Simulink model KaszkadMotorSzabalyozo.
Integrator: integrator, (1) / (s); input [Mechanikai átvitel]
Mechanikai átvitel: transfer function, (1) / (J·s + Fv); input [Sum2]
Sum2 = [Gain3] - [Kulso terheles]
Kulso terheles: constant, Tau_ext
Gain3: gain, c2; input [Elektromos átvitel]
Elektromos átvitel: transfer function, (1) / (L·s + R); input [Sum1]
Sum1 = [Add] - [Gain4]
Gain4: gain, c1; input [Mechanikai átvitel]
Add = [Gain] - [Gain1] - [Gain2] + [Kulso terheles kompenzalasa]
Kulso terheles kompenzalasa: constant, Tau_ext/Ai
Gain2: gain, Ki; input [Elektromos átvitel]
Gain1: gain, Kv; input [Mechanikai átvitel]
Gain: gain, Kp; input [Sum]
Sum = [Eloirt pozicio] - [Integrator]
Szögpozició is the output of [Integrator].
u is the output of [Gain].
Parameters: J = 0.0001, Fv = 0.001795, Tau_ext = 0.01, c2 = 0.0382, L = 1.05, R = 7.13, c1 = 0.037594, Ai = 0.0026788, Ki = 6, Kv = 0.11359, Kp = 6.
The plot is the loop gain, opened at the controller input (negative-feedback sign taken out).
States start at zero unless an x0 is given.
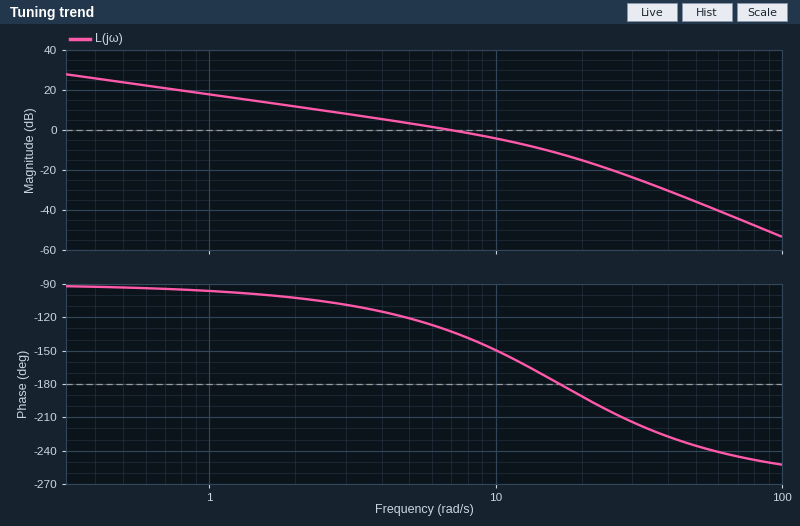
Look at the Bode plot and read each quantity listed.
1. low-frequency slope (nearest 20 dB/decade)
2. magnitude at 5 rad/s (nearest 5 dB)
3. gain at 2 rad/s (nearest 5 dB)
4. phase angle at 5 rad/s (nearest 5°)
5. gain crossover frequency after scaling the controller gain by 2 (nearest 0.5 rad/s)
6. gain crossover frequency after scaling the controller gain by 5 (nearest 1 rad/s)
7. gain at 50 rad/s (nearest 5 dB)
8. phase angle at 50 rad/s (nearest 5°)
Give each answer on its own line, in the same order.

-20 dB/decade
5 dB
10 dB
-120°
11.5 rad/s
19 rad/s
-35 dB
-235°
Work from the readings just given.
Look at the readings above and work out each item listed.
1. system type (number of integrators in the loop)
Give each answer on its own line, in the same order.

1
